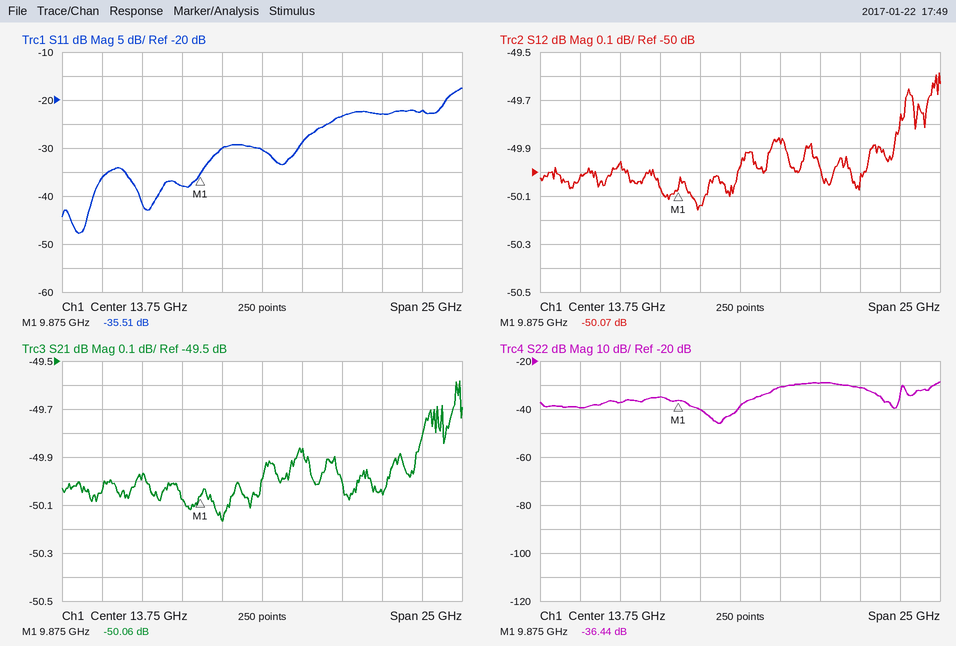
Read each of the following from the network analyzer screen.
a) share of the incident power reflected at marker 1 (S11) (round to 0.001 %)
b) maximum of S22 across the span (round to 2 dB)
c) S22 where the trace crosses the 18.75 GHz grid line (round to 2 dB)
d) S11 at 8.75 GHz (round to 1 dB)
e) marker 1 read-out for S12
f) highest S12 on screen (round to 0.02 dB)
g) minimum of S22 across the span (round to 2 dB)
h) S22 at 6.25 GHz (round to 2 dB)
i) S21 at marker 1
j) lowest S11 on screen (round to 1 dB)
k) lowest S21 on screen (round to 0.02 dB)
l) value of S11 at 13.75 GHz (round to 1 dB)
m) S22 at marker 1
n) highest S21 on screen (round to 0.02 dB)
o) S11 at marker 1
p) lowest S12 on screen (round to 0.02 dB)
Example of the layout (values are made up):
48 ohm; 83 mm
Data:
0.028 %; -28 dB; -30 dB; -38 dB; -50.07 dB; -49.58 dB; -46 dB; -38 dB; -50.06 dB; -48 dB; -50.16 dB; -30 dB; -36.44 dB; -49.58 dB; -35.51 dB; -50.16 dB
